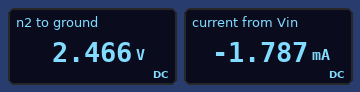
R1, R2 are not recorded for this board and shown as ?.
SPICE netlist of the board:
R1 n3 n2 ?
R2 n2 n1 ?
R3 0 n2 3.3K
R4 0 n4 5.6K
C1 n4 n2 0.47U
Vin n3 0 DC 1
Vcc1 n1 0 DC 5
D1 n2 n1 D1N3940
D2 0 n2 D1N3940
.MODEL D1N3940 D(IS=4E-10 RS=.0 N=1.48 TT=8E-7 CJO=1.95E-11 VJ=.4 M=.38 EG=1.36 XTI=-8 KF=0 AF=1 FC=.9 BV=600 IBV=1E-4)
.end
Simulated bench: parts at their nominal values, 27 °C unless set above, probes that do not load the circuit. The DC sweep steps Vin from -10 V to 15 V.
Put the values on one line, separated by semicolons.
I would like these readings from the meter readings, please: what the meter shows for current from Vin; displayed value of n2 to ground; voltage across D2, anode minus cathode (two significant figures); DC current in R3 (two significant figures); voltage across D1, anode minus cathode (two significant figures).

-1.787 mA; 2.466 V; -2.5 V; 750 µA; -2.5 V
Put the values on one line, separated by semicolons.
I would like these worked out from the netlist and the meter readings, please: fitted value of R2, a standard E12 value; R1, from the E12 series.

1 kΩ; 820 Ω
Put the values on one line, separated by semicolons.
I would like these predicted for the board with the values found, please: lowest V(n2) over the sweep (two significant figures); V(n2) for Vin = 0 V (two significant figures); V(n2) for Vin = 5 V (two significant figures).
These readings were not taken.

-630 mV; 2.0 V; 4.4 V
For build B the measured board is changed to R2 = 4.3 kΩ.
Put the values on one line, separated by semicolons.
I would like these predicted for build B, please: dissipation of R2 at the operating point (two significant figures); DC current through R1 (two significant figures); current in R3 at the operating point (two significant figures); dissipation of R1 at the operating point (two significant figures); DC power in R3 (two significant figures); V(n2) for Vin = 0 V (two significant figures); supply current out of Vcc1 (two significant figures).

3.1 mW; 440 µA; 410 µA; 160 µW; 560 µW; 660 mV; 850 µA
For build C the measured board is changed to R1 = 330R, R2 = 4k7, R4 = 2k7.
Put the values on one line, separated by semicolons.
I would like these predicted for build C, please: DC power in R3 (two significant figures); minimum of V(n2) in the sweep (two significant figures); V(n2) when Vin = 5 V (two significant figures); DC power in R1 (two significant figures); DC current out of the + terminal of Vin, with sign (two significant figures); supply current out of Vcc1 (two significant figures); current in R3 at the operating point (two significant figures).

400 µW; -690 mV; 4.6 V; 72 µW; -470 µA; 820 µA; 350 µA
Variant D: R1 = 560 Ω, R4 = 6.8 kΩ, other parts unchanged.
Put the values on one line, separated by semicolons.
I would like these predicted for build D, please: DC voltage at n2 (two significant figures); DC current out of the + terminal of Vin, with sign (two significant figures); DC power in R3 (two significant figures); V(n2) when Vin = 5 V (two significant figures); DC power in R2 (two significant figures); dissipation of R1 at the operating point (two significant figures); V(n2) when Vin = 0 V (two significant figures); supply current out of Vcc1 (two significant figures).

2.2 V; -2.1 mA; 1.5 mW; 4.5 V; 7.9 mW; 2.6 mW; 1.6 V; 2.8 mA
